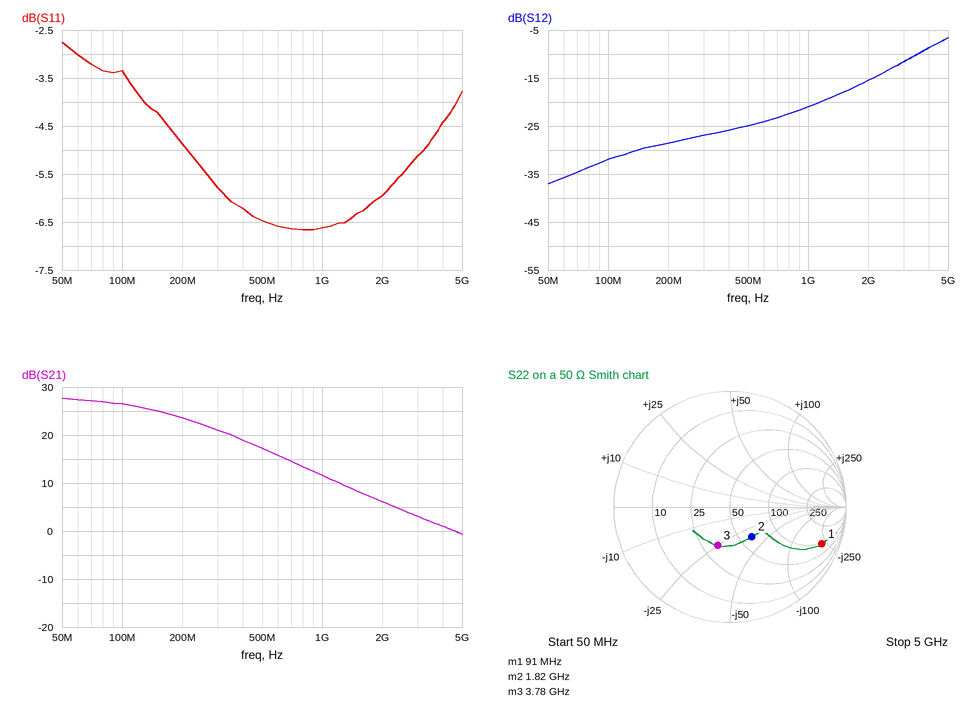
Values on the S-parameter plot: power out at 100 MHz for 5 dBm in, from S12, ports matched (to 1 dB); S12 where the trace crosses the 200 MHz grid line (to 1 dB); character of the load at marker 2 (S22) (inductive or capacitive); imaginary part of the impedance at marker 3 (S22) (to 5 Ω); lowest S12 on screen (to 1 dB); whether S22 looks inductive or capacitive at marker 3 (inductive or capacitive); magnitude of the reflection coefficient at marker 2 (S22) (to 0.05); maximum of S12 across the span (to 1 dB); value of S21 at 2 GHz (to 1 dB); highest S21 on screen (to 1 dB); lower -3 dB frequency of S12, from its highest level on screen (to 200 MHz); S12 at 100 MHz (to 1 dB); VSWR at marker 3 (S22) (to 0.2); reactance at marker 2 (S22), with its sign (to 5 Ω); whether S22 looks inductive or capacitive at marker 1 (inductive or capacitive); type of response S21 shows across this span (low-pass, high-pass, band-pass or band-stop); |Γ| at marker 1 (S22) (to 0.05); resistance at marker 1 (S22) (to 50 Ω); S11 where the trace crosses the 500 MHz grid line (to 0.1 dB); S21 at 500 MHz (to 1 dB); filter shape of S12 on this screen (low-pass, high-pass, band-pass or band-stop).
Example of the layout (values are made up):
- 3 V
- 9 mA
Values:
- -27 dBm
- -29 dB
- capacitive
- -25 Ω
- -37 dB
- capacitive
- 0.30
- -7 dB
- 6 dB
- 28 dB
- 3.6 GHz
- -32 dB
- 2.0
- -35 Ω
- capacitive
- low-pass
- 0.85
- 100 Ω
- -6.5 dB
- 17 dB
- high-pass
